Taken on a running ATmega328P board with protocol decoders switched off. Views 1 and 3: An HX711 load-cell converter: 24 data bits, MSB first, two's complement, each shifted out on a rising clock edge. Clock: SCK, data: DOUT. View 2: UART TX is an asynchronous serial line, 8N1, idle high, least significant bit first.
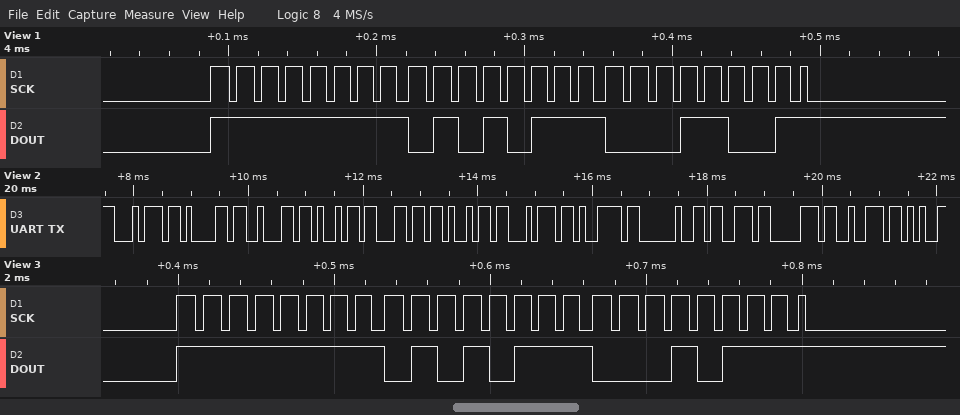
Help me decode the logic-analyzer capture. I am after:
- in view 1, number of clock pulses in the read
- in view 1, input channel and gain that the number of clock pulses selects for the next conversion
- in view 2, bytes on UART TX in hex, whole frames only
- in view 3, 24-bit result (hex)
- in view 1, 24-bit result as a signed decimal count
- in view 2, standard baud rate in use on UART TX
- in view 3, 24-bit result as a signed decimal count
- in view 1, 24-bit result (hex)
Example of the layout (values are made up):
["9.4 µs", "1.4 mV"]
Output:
["25", "channel A, gain 128", "74 61 62 69 6C 69 74 79 20 73 70 72", "0xFF5717", "-43239", "9600 baud", "-43241", "0xFF5719"]
